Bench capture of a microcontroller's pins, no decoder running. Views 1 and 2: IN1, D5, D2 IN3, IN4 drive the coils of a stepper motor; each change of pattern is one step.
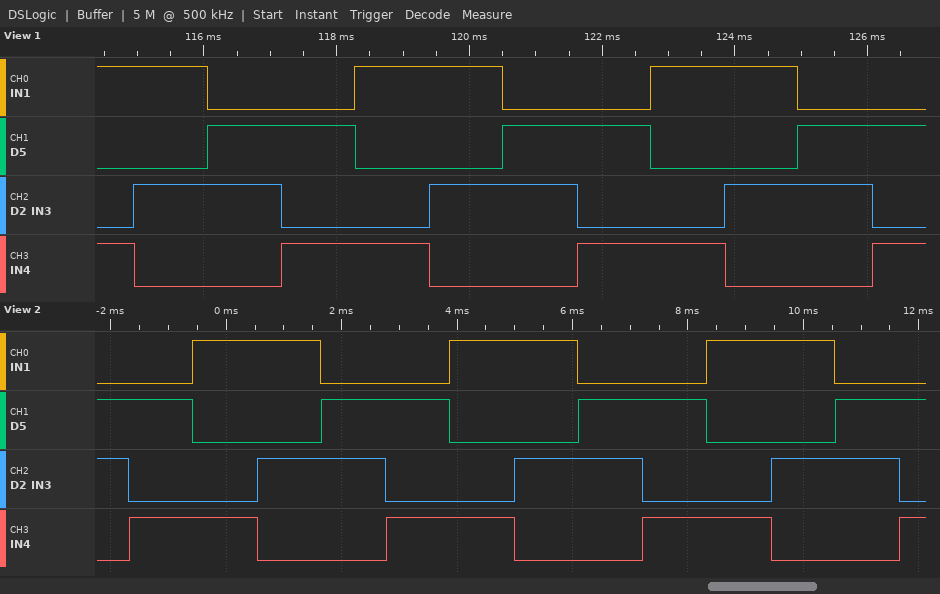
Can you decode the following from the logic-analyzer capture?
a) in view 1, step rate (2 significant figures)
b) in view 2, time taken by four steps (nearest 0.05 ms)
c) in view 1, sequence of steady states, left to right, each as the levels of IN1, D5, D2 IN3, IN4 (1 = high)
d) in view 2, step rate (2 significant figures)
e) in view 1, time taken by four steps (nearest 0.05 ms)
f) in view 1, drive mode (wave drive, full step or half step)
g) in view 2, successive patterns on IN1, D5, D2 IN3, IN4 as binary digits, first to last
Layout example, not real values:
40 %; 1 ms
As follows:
900 steps/s; 4.45 ms; 1001 1010 0110 0101 1001 1010 0110 0101 1001 1010 0110 0101; 900 steps/s; 4.45 ms; full step; 0110 0101 1001 1010 0110 0101 1001 1010 0110 0101 1001 1010 0110 0101
